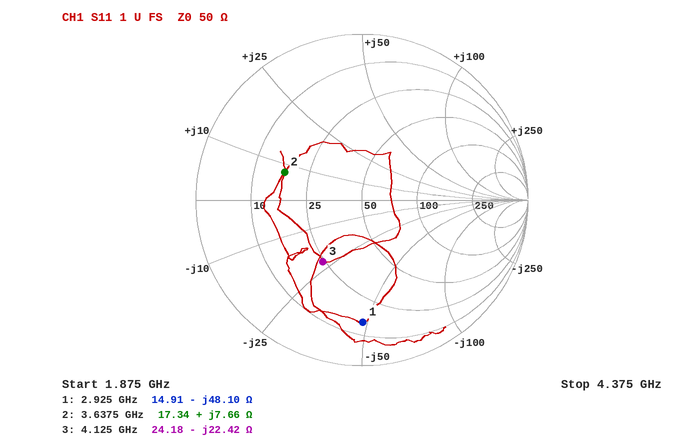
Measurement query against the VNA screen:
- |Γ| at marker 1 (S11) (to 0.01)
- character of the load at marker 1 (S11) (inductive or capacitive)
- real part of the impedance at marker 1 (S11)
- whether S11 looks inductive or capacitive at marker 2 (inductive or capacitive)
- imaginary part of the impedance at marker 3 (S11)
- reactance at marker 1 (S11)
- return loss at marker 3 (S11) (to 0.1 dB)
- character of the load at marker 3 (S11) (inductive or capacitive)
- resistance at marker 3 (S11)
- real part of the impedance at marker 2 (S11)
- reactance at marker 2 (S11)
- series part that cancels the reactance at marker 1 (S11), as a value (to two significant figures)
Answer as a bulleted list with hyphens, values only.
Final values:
- 0.74
- capacitive
- 14.91 Ω
- inductive
- -22.42 Ω
- -48.10 Ω
- 7.1 dB
- capacitive
- 24.18 Ω
- 17.34 Ω
- +7.66 Ω
- 2.6 nH
